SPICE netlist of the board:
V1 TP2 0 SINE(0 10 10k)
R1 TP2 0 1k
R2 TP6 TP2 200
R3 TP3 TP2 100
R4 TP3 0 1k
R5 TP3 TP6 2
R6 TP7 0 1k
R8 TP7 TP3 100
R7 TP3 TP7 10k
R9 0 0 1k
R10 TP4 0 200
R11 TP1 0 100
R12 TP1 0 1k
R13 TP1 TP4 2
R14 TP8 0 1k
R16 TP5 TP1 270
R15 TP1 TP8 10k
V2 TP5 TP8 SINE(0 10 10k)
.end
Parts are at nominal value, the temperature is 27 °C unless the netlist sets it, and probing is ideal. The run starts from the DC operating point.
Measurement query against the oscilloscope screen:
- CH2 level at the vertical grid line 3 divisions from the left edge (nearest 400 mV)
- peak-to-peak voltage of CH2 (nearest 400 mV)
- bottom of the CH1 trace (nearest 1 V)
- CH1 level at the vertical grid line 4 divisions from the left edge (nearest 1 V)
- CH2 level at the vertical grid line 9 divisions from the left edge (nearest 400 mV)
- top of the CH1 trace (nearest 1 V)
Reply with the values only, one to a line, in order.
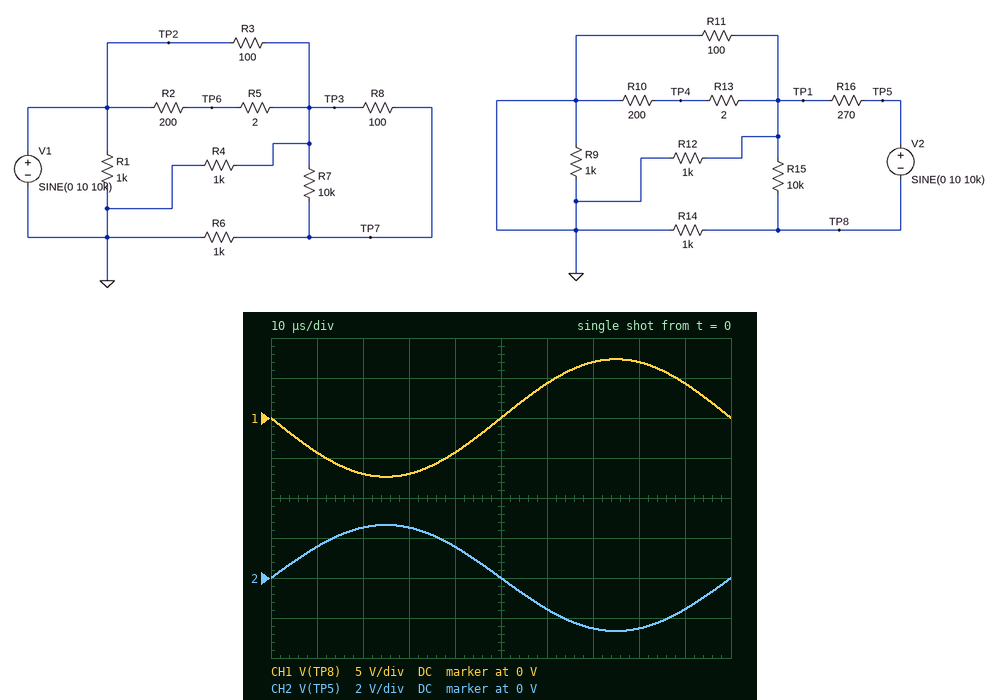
2.4 V
5.2 V
-7 V
-4 V
-1.6 V
7 V
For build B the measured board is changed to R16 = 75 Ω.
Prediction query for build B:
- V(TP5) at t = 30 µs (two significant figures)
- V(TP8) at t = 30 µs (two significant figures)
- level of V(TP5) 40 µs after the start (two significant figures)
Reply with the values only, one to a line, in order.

1.2 V
-8.3 V
750 mV
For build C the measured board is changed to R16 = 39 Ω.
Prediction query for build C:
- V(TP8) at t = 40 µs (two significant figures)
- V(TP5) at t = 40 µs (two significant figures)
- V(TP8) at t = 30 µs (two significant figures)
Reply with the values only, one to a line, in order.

-5.3 V
560 mV
-8.6 V
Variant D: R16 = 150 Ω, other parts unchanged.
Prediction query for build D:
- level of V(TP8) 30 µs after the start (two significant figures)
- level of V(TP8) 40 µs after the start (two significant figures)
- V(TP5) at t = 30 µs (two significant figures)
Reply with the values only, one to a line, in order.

-7.7 V
-4.8 V
1.8 V
